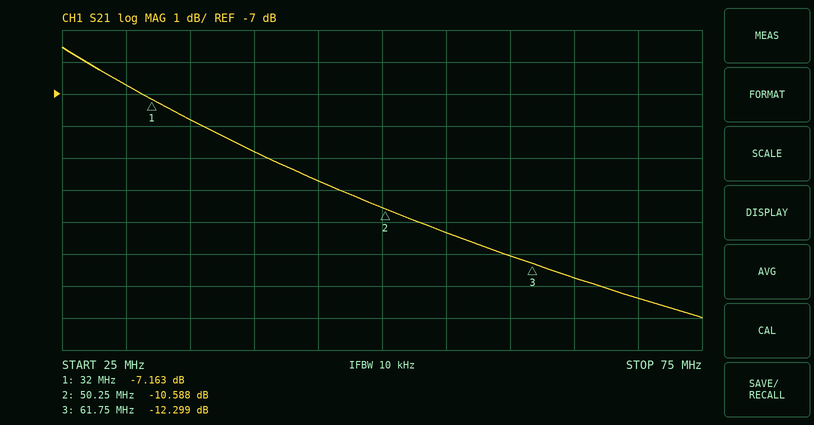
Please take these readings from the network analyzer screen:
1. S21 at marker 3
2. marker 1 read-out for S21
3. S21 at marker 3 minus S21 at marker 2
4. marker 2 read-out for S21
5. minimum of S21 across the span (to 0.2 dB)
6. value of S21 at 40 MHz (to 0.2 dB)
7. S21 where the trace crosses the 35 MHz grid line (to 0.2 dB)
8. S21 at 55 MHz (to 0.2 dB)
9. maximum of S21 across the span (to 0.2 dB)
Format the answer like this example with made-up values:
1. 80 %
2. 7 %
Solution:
1. -12.299 dB
2. -7.163 dB
3. -1.711 dB
4. -10.588 dB
5. -14.0 dB
6. -8.8 dB
7. -7.8 dB
8. -11.4 dB
9. -5.6 dB
